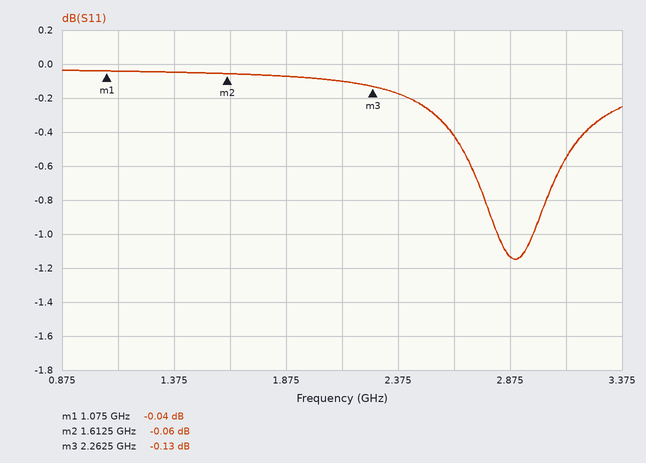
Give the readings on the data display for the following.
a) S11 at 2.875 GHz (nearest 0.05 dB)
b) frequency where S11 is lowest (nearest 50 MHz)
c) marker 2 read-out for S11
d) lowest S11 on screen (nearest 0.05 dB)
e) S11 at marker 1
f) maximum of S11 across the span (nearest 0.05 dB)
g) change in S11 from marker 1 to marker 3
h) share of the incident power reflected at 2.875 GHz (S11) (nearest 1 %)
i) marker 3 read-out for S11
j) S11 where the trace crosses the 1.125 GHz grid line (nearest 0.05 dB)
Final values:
-1.15 dB
2.90 GHz
-0.06 dB
-1.15 dB
-0.04 dB
-0.05 dB
-0.09 dB
77 %
-0.13 dB
-0.05 dB
